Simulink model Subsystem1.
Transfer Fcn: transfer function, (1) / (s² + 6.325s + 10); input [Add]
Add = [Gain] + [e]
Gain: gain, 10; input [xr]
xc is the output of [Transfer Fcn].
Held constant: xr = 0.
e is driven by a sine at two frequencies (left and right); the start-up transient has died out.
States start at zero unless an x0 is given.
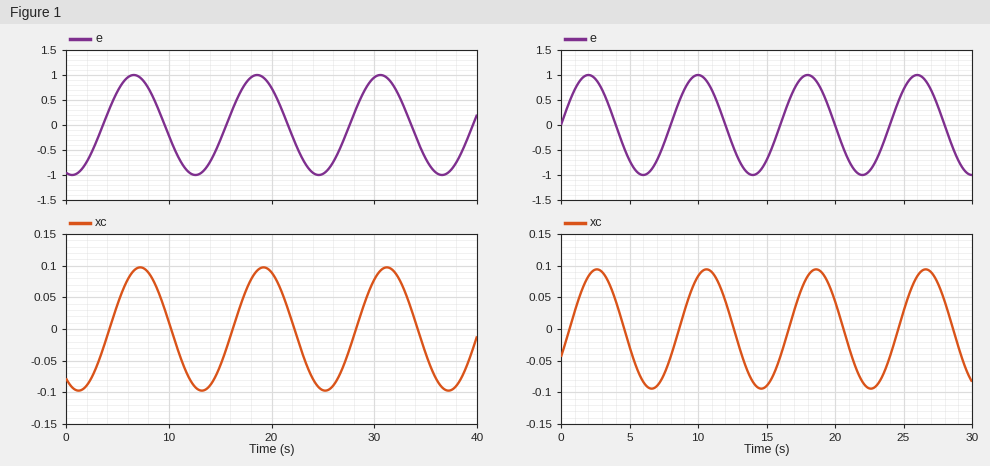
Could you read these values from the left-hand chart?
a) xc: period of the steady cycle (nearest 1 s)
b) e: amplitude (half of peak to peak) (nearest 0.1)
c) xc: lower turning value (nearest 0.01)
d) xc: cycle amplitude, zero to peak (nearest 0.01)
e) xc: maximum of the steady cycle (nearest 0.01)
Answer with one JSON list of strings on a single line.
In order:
["12 s", "1.0", "-0.10", "0.10", "0.10"]
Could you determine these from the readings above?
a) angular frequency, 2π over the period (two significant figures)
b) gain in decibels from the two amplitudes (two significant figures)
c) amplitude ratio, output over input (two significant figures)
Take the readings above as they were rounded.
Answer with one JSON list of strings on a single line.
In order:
["0.52 rad/s", "-20 dB", "0.10"]
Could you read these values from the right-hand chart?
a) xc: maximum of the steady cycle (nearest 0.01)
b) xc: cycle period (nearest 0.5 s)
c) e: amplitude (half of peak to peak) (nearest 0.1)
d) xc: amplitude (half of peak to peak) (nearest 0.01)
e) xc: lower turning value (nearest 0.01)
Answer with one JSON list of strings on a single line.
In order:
["0.09", "8.0 s", "1.0", "0.09", "-0.09"]
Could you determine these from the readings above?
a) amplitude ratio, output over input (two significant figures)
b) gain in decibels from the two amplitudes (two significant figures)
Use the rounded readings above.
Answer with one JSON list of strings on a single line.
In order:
["0.090", "-21 dB"]
